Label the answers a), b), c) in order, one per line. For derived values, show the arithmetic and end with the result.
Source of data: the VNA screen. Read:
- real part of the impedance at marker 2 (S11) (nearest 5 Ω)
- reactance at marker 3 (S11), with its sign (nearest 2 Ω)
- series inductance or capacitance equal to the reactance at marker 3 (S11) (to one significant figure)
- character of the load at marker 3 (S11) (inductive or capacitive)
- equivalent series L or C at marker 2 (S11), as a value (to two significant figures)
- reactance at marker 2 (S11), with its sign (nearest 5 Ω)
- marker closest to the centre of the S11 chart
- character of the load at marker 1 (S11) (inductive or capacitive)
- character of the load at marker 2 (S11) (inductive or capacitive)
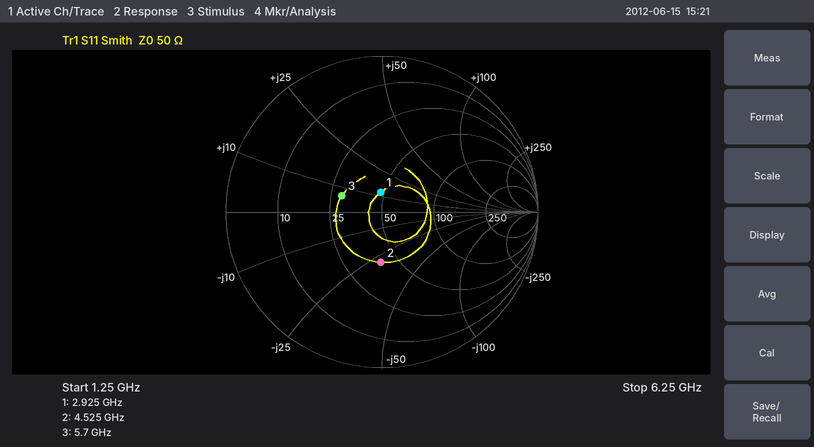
a) 40 Ω
b) +6 Ω
c) L = 6 Ω/(2π × 5.7 GHz) ≈ 168 pH, so 200 pH to one significant figure
d) inductive
e) C = 1/(2π × 4.525 GHz × 30 Ω) ≈ 1.2 pF
f) -30 Ω
g) marker 1
h) inductive
i) capacitive
